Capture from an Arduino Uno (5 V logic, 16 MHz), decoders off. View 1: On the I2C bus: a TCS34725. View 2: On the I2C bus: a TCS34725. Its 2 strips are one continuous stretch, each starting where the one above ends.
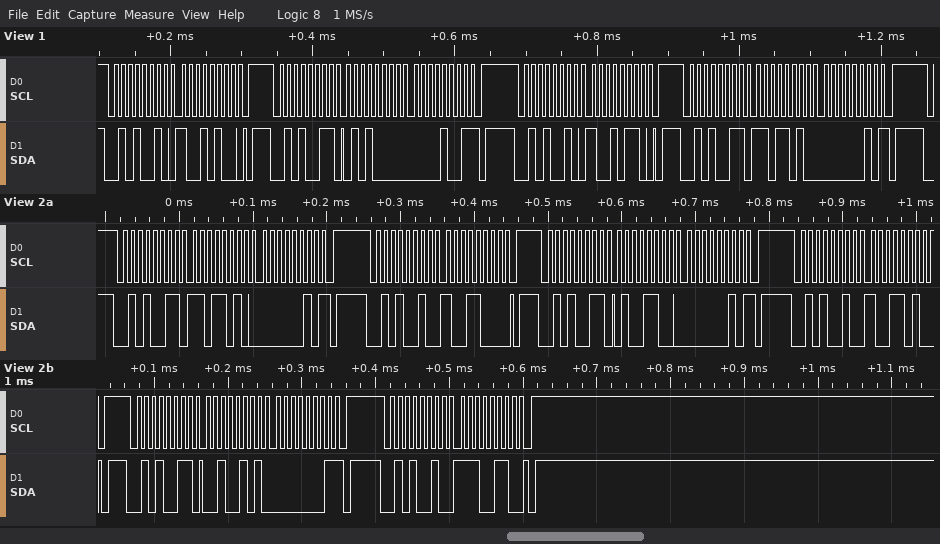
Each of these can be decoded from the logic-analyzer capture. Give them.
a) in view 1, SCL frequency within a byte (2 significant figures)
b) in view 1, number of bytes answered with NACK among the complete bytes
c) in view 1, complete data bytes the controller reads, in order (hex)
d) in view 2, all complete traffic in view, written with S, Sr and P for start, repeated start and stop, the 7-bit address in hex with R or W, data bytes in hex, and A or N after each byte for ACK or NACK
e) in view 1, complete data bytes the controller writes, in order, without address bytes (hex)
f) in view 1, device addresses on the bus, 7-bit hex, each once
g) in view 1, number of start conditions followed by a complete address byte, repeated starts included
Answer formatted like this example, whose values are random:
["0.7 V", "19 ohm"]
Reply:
["100 kHz", "2", "50 09 DA 02", "S 29R A DA A 02 N P S 29W A 98 A P S 29R A 4C A 02 N P S 29W A 9A A P S 29R A 25 A 01 N P S 29W A E6 A P", "94 96", "0x29", "4"]
